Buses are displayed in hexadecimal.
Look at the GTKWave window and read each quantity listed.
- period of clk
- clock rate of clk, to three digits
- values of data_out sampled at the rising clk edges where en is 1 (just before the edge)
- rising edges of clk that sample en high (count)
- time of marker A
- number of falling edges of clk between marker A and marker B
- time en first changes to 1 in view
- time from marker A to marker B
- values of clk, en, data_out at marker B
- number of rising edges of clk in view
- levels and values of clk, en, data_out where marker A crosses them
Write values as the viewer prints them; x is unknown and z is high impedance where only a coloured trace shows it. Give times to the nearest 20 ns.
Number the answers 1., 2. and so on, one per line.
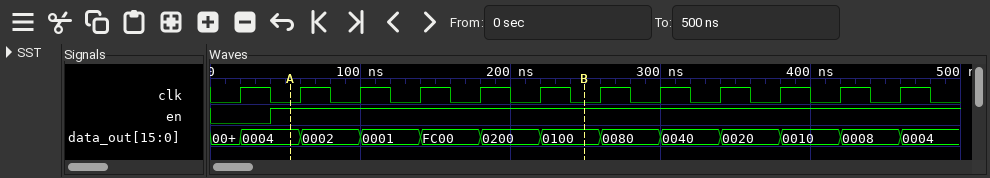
1. 40 ns
2. 25.0 MHz
3. 0004, 0002, 0001, FC00, 0200, 0100, 0080, 0040, 0020, 0010, 0008
4. 11
5. 60 ns
6. 5
7. 40 ns
8. 200 ns
9. clk=0, en=1, data_out=0100
10. 12
11. clk=0, en=1, data_out=0004
